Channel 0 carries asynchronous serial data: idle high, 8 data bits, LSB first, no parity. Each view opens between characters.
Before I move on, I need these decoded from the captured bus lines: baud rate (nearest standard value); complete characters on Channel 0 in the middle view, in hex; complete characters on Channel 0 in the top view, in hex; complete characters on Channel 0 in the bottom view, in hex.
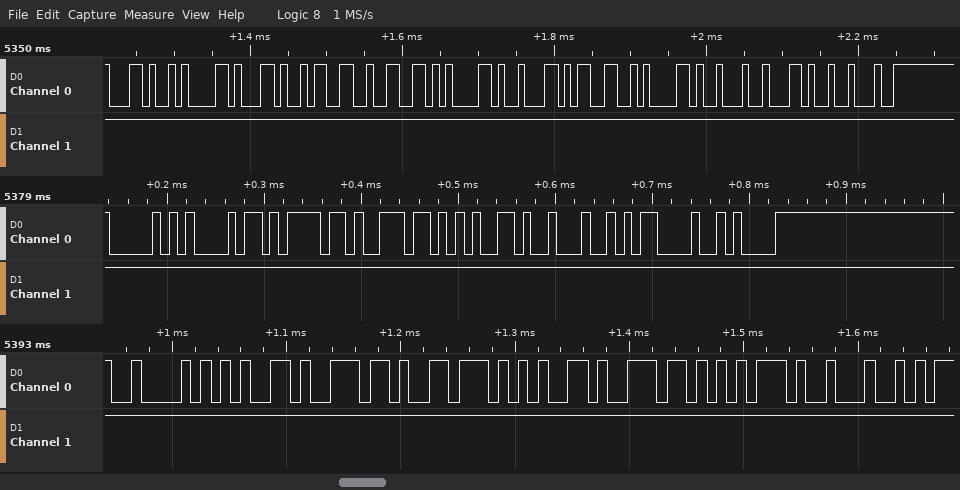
115200 baud
50, 68, 6F, 6E, 65, 22, 0D, 0A
2C, 61, 2C, 33, 66, 61, 62, 33, 61, 22, 2C, 22
42, 65, 6E, 76, 65, 6E, 75, 22
